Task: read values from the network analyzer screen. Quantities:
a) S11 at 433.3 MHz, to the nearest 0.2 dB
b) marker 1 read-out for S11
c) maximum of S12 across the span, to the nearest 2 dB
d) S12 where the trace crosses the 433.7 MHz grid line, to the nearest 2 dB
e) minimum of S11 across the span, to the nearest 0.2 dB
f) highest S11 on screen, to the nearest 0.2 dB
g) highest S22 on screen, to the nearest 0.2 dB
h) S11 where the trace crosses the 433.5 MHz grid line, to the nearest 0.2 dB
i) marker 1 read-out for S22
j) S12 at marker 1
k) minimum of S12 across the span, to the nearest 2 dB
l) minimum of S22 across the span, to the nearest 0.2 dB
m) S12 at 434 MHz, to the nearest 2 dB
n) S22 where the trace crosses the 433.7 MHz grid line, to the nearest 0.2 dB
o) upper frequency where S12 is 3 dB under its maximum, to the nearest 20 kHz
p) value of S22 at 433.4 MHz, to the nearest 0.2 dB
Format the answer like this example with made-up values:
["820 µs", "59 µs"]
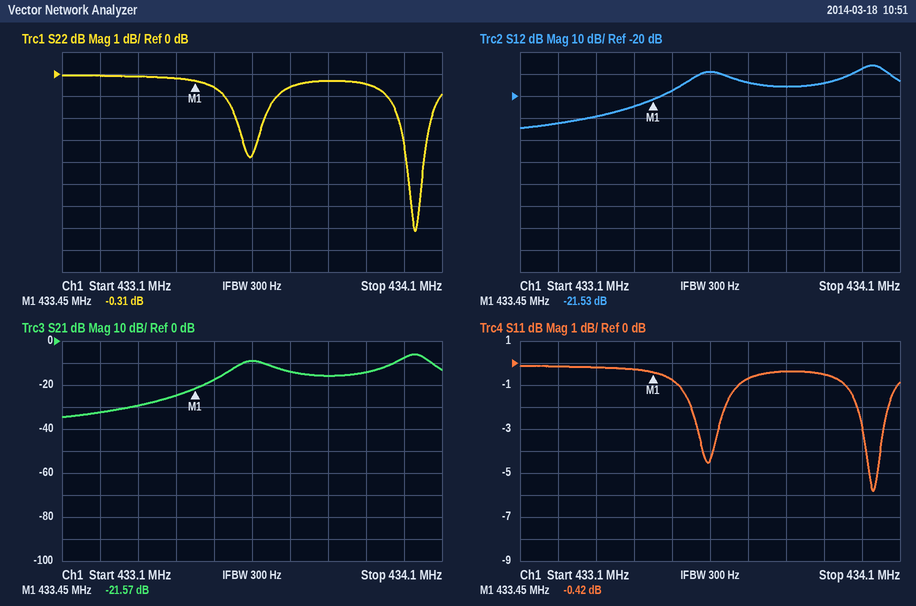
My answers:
["-0.2 dB", "-0.42 dB", "-6 dB", "-14 dB", "-5.8 dB", "-0.2 dB", "0.0 dB", "-0.8 dB", "-0.31 dB", "-21.53 dB", "-34 dB", "-7.2 dB", "-8 dB", "-0.6 dB", "434.06 MHz", "-0.2 dB"]
